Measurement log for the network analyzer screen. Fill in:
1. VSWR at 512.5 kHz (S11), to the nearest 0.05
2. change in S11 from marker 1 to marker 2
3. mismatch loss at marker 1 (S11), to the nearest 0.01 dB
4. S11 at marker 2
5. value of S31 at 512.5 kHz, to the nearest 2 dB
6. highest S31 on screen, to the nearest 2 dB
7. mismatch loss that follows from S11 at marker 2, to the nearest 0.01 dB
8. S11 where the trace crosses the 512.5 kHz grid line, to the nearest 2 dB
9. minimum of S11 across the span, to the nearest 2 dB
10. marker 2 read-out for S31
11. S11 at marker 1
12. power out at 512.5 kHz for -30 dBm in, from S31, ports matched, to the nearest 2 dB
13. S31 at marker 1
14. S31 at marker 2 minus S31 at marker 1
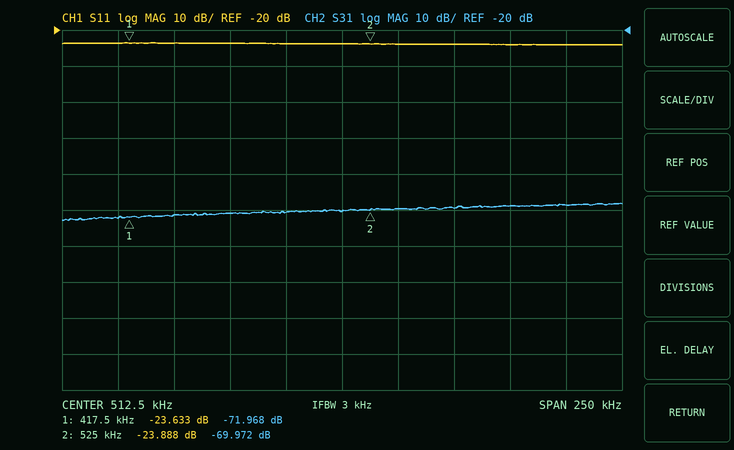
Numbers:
1.15
-0.255 dB
0.02 dB
-23.888 dB
-70 dB
-68 dB
0.02 dB
-24 dB
-24 dB
-69.972 dB
-23.633 dB
-100 dBm
-71.968 dB
1.996 dB
